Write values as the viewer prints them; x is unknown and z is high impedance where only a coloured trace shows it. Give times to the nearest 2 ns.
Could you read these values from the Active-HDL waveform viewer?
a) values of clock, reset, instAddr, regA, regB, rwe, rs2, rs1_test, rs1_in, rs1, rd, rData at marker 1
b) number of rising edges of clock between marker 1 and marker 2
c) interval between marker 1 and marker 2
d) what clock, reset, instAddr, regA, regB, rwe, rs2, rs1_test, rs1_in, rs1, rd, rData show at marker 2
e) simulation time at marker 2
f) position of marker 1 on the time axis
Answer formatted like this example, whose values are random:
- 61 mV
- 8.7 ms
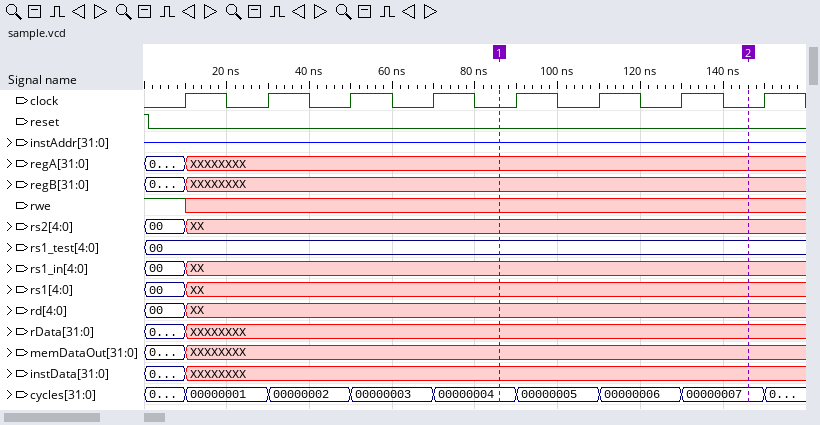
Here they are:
- clock=0, reset=0, instAddr=z, regA=XXXXXXXX, regB=XXXXXXXX, rwe=x, rs2=XX, rs1_test=00, rs1_in=XX, rs1=XX, rd=XX, rData=XXXXXXXX
- 3
- 60 ns
- clock=0, reset=0, instAddr=z, regA=XXXXXXXX, regB=XXXXXXXX, rwe=x, rs2=XX, rs1_test=00, rs1_in=XX, rs1=XX, rd=XX, rData=XXXXXXXX
- 146 ns
- 86 ns
